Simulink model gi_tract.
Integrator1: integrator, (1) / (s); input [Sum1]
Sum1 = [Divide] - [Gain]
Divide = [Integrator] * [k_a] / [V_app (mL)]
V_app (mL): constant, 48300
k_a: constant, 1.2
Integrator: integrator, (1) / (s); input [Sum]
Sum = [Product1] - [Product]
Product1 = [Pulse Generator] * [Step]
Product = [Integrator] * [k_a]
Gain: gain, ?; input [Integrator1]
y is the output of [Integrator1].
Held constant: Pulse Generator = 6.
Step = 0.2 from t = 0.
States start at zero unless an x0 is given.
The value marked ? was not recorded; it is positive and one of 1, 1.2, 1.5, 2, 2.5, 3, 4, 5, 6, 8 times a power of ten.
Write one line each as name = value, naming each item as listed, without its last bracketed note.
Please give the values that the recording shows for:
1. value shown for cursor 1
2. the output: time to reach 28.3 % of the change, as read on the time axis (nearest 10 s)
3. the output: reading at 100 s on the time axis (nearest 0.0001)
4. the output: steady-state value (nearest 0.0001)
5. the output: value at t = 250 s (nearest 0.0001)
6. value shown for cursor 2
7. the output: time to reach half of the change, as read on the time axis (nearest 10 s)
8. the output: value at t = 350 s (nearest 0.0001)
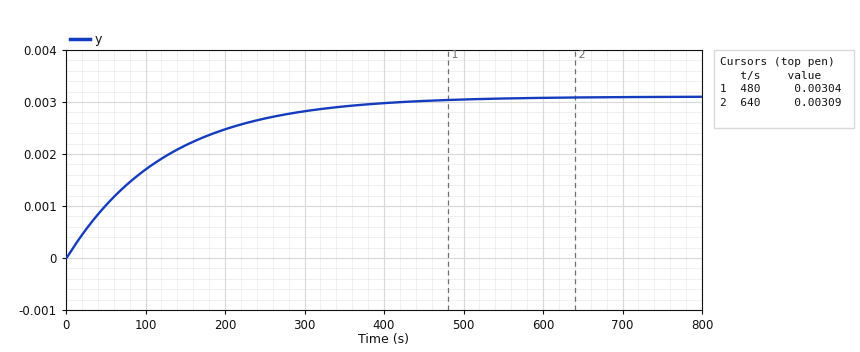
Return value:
value shown for cursor 1 = 0.00304
the output: time to reach 28.3 % of the change, as read on the time axis = 40 s
the output: reading at 100 s on the time axis = 0.0017
the output: steady-state value = 0.0031
the output: value at t = 250 s = 0.0027
value shown for cursor 2 = 0.00309
the output: time to reach half of the change, as read on the time axis = 90 s
the output: value at t = 350 s = 0.0029
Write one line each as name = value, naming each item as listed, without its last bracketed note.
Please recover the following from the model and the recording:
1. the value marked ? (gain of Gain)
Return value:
the value marked ? = 0.008
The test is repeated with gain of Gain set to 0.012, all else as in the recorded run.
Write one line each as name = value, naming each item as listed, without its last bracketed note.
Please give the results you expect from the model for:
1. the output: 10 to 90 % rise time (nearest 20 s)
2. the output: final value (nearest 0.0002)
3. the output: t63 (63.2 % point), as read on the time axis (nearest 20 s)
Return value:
the output: 10 to 90 % rise time = 180 s
the output: final value = 0.0020
the output: t63 (63.2 % point), as read on the time axis = 80 s
